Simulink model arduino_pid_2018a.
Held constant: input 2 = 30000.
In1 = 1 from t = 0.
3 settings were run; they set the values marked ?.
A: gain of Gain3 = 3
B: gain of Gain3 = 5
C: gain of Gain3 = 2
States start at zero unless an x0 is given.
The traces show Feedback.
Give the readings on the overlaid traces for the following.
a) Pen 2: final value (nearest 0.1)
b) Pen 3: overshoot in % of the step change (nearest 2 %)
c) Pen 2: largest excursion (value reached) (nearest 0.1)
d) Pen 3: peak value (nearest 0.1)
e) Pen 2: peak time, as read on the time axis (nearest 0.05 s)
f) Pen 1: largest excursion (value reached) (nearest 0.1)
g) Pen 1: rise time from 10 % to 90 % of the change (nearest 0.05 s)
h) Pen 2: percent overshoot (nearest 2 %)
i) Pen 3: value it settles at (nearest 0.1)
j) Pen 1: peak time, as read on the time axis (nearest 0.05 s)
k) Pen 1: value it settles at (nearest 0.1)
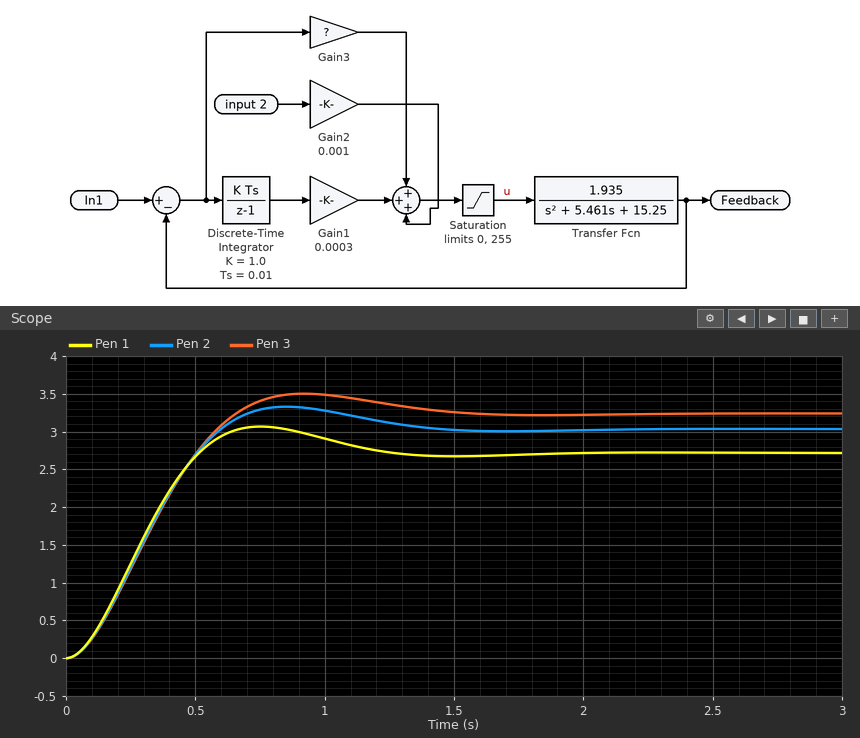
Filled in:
3.0
8 %
3.3
3.5
0.85 s
3.1
0.35 s
10 %
3.2
0.75 s
2.7
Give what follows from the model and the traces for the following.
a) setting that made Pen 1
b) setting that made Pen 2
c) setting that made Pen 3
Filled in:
B
A
C
